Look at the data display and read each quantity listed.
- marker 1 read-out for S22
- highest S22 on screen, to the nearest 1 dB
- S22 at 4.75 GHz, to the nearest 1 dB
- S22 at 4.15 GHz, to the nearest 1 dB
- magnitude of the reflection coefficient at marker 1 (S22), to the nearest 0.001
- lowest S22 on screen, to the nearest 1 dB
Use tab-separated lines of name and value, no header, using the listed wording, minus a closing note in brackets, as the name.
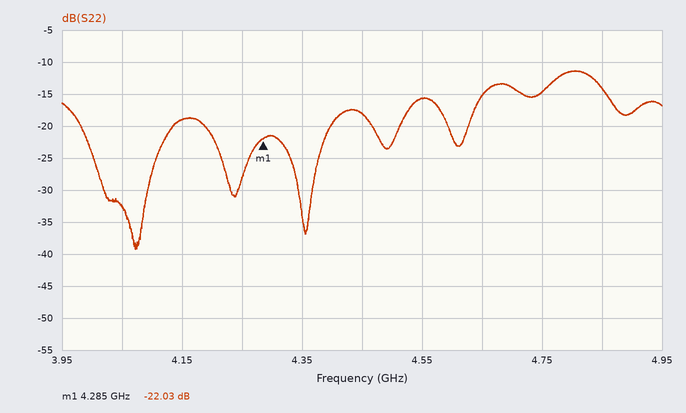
marker 1 read-out for S22	-22.03 dB
highest S22 on screen, to the nearest 1 dB	-11 dB
S22 at 4.75 GHz, to the nearest 1 dB	-15 dB
S22 at 4.15 GHz, to the nearest 1 dB	-19 dB
magnitude of the reflection coefficient at marker 1 (S22), to the nearest 0.001	0.079
lowest S22 on screen, to the nearest 1 dB	-39 dB
